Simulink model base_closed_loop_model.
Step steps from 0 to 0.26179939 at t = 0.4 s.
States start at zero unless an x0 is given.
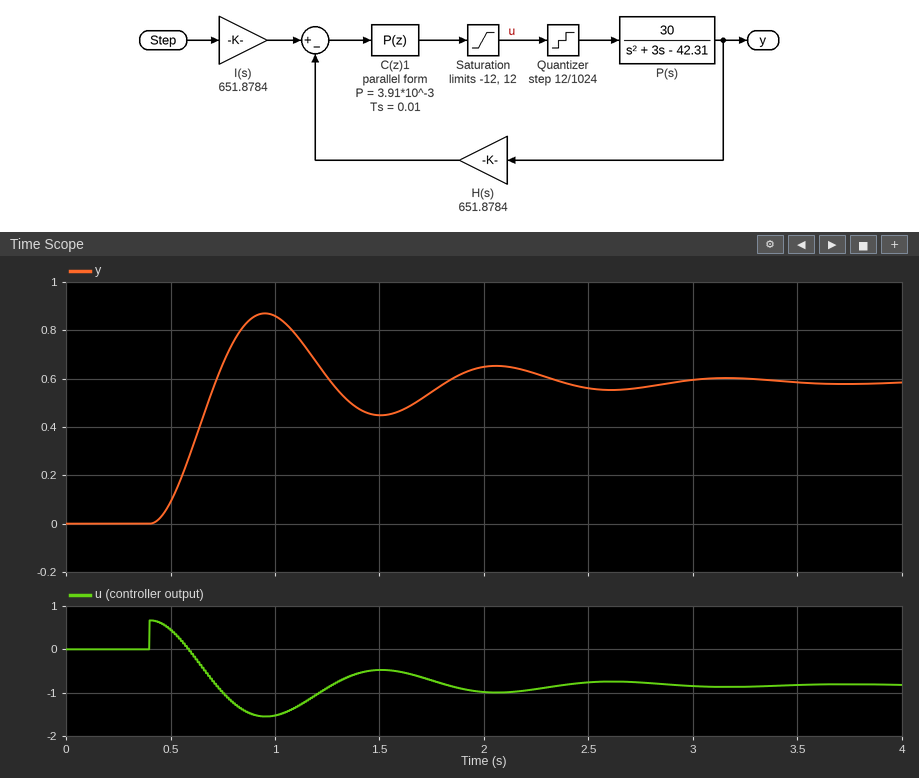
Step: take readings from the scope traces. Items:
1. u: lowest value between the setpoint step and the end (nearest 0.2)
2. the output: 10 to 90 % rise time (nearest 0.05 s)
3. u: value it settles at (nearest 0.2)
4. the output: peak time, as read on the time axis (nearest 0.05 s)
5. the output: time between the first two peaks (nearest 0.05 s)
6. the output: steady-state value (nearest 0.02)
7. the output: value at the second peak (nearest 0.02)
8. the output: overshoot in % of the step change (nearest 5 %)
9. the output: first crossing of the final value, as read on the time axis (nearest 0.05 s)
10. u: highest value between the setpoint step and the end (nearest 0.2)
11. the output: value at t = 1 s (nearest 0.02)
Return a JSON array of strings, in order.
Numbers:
["-1.6", "0.20 s", "-0.8", "0.95 s", "1.10 s", "0.58", "0.66", "50 %", "0.70 s", "0.6", "0.86"]
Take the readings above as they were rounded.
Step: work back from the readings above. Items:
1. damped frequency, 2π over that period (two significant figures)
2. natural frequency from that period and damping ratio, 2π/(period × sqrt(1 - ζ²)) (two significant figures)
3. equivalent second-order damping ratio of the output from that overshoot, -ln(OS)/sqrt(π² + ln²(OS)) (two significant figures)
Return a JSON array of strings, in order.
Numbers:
["5.7 rad/s", "5.9 rad/s", "0.22"]
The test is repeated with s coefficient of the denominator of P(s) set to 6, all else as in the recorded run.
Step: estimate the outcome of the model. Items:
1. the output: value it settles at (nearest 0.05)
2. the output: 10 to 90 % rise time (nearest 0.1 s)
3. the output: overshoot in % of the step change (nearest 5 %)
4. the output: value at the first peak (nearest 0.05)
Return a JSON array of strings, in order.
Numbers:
["0.60", "0.3 s", "20 %", "0.70"]
